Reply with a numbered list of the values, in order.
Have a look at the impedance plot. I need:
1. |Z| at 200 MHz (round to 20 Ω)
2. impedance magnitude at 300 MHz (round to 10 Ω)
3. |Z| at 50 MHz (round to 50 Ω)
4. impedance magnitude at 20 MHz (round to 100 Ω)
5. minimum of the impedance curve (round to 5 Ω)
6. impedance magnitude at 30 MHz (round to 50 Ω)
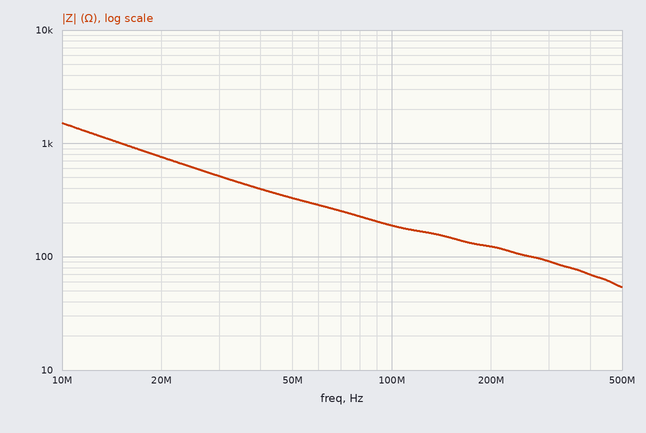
1. 120 Ω
2. 90 Ω
3. 350 Ω
4. 800 Ω
5. 55 Ω
6. 500 Ω
